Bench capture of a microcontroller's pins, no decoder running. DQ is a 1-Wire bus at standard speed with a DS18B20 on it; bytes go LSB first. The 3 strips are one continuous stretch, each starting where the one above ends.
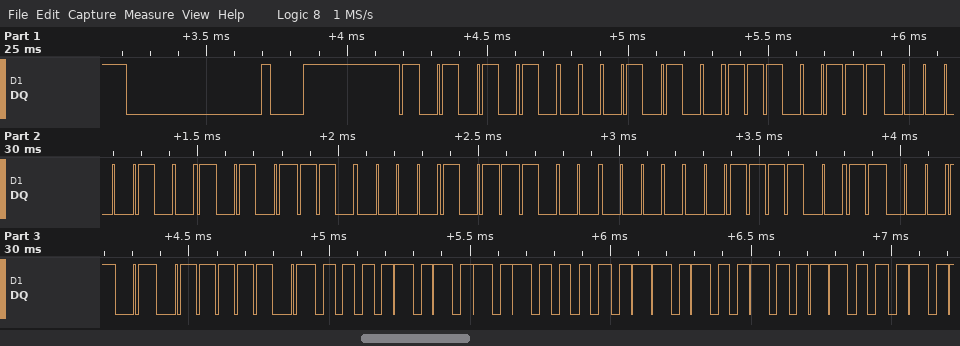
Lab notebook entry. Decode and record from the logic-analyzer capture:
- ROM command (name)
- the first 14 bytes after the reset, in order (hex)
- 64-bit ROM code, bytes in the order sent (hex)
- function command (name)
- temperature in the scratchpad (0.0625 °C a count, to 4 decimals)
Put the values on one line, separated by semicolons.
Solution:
Match ROM; 55 28 E7 20 75 D0 01 3C A3 BE 50 05 4B 46; 28 E7 20 75 D0 01 3C A3; Read Scratchpad; 85.0000 °C
